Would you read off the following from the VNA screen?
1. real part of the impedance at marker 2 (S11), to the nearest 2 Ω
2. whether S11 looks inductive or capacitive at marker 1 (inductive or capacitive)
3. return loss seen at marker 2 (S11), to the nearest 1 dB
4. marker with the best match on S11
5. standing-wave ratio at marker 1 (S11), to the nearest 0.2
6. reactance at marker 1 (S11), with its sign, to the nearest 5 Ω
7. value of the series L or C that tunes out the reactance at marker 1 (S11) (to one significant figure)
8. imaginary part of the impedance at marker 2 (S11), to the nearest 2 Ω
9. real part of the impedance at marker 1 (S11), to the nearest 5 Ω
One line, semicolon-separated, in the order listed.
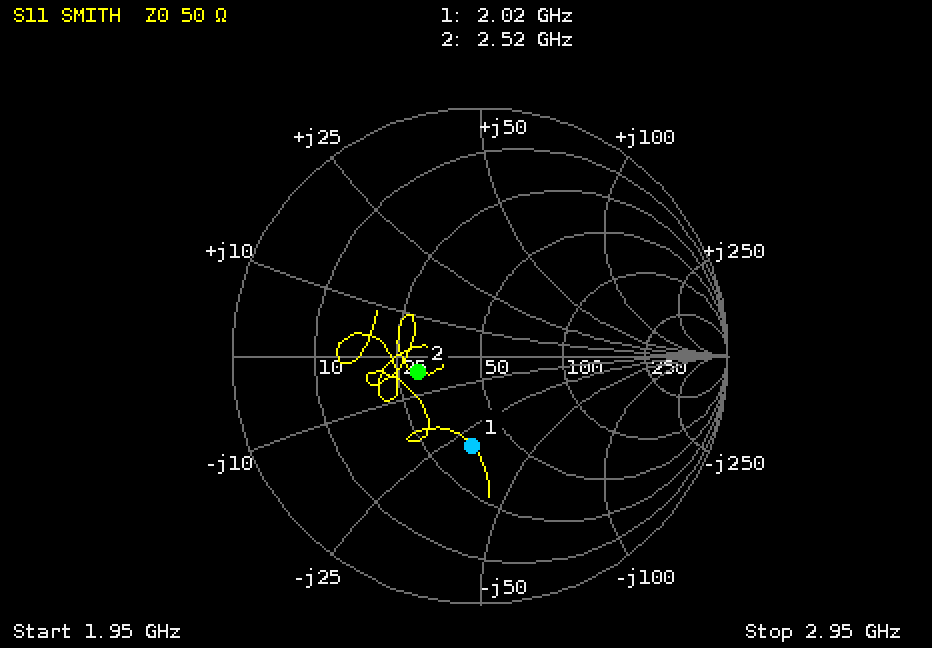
30 Ω; capacitive; 12 dB; marker 2; 2.2; -30 Ω; 2 nH; -4 Ω; 35 Ω
